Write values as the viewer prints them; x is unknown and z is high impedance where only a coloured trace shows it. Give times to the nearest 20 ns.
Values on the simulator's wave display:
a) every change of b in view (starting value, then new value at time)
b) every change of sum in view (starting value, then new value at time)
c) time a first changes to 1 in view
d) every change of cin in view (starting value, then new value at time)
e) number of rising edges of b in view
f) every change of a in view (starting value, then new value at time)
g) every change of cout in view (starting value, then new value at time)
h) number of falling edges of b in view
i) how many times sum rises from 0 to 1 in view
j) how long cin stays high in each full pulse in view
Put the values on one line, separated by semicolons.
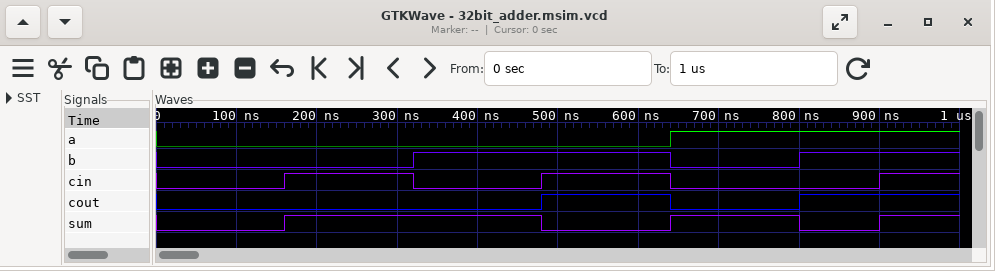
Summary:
0, 1 at 320 ns, 0 at 640 ns, 1 at 800 ns; 0, 1 at 160 ns, 0 at 480 ns, 1 at 640 ns, 0 at 800 ns, 1 at 900 ns; 640 ns; 0, 1 at 160 ns, 0 at 320 ns, 1 at 480 ns, 0 at 640 ns, 1 at 900 ns; 2; 0, 1 at 640 ns; 0, 1 at 480 ns, 0 at 640 ns, 1 at 800 ns; 1; 3; 160 ns, 160 ns
